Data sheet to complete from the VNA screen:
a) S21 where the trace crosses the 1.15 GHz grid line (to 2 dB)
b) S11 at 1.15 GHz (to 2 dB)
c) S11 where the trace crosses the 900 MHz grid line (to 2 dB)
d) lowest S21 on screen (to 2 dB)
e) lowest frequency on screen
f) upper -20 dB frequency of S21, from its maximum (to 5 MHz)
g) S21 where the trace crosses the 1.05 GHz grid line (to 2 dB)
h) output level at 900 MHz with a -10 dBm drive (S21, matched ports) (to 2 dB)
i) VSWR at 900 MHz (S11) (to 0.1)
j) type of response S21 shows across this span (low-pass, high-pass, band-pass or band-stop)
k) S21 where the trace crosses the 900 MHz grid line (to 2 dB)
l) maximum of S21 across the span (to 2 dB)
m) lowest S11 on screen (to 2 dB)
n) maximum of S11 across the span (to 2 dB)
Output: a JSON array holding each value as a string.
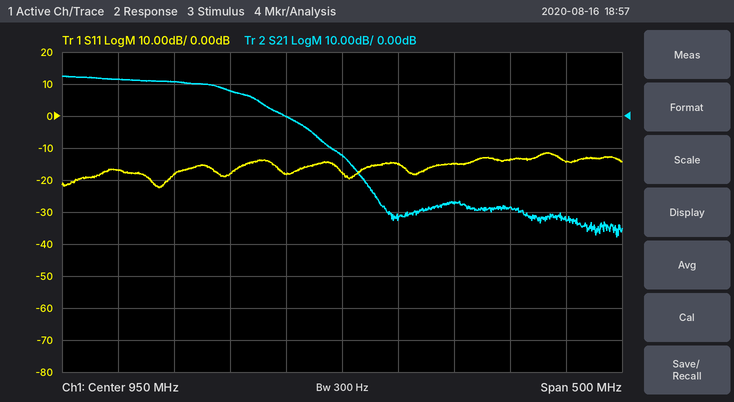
["-32 dB", "-14 dB", "-18 dB", "-38 dB", "700 MHz", "930 MHz", "-28 dB", "-10 dBm", "1.3", "low-pass", "0 dB", "12 dB", "-22 dB", "-12 dB"]
